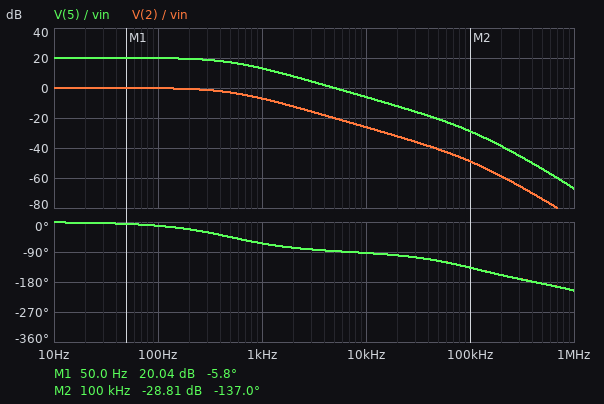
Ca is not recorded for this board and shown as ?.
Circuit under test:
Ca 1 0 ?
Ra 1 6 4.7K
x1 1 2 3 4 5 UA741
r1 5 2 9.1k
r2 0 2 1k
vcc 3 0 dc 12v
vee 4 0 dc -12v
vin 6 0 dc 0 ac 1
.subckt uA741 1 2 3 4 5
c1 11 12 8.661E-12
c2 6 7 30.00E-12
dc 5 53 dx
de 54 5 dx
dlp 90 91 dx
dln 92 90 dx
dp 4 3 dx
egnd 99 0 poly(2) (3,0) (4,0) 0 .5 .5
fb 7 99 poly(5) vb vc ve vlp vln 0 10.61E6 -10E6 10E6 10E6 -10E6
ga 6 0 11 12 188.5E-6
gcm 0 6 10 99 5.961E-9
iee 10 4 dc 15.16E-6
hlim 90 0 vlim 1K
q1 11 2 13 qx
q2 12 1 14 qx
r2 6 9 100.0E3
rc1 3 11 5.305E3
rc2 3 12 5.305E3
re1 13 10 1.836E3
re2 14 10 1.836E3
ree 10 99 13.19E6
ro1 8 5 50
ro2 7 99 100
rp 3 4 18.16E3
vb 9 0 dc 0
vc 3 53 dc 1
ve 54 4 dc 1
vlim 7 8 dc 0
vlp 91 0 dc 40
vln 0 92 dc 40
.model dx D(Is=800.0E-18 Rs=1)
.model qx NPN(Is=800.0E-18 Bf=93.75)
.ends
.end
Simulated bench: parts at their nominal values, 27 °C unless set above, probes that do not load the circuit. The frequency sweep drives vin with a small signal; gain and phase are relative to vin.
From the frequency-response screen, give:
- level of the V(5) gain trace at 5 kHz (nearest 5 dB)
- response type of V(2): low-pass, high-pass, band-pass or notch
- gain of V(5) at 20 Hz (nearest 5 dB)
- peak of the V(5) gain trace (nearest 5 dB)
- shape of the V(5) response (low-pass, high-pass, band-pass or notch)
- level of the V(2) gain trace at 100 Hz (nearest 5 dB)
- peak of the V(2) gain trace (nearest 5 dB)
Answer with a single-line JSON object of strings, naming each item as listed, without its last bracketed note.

{"level of the V(5) gain trace at 5 kHz": "0 dB", "response type of V(2): low-pass, high-pass, band-pass or notch": "low-pass", "gain of V(5) at 20 Hz": "20 dB", "peak of the V(5) gain trace": "20 dB", "shape of the V(5) response": "low-pass", "level of the V(2) gain trace at 100 Hz": "0 dB", "peak of the V(2) gain trace": "0 dB"}
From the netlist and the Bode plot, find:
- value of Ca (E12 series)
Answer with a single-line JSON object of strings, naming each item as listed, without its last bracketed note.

{"value of Ca": "68 nF"}
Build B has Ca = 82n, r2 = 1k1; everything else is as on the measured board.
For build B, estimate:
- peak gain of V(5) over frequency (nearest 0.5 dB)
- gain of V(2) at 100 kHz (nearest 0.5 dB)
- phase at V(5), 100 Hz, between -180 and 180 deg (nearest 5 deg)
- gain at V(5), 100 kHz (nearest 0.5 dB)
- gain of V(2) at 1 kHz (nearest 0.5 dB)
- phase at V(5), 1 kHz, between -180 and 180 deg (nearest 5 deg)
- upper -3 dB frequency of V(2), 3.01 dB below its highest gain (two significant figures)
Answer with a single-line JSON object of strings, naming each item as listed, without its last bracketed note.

{"peak gain of V(5) over frequency": "19.5 dB", "gain of V(2) at 100 kHz": "-50.0 dB", "phase at V(5), 100 Hz, between -180 and 180 deg": "-15 deg", "gain at V(5), 100 kHz": "-31.0 dB", "gain of V(2) at 1 kHz": "-8.5 dB", "phase at V(5), 1 kHz, between -180 and 180 deg": "-70 deg", "upper -3 dB frequency of V(2), 3.01 dB below its highest gain": "410 Hz"}
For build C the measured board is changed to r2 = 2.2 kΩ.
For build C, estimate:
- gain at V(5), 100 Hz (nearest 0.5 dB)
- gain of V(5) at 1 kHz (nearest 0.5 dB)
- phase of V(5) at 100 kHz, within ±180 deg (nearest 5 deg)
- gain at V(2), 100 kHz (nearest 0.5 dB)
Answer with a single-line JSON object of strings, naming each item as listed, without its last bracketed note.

{"gain at V(5), 100 Hz": "14.0 dB", "gain of V(5) at 1 kHz": "7.0 dB", "phase of V(5) at 100 kHz, within ±180 deg": "-120 deg", "gain at V(2), 100 kHz": "-47.0 dB"}
